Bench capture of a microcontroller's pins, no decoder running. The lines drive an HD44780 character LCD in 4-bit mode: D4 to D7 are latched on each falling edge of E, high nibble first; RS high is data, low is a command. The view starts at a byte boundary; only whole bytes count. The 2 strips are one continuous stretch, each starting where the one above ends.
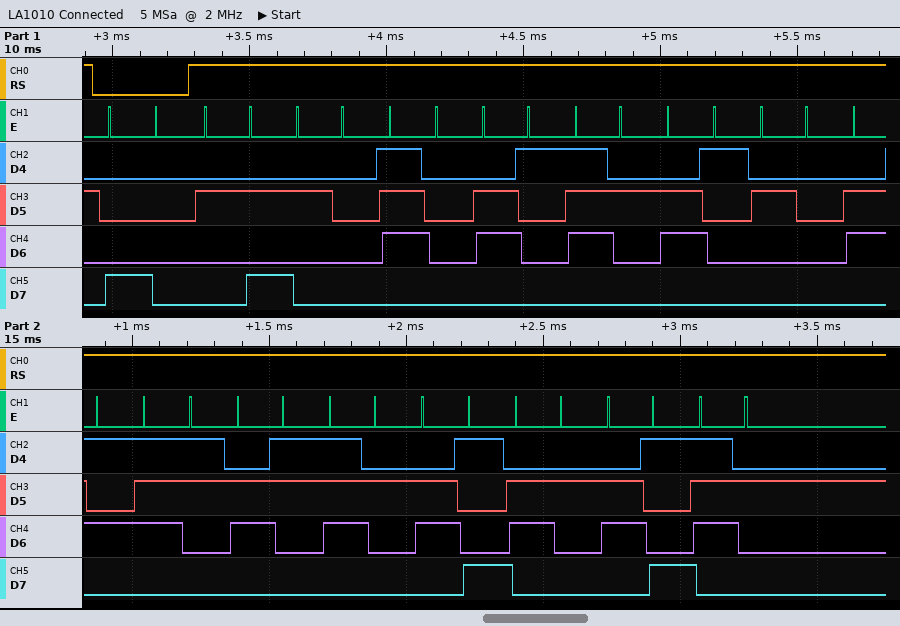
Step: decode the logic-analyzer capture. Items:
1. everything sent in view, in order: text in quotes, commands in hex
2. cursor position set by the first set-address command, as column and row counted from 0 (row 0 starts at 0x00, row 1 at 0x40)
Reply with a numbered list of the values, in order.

1. 0x80 "* para escribir"
2. column 0, row 0
